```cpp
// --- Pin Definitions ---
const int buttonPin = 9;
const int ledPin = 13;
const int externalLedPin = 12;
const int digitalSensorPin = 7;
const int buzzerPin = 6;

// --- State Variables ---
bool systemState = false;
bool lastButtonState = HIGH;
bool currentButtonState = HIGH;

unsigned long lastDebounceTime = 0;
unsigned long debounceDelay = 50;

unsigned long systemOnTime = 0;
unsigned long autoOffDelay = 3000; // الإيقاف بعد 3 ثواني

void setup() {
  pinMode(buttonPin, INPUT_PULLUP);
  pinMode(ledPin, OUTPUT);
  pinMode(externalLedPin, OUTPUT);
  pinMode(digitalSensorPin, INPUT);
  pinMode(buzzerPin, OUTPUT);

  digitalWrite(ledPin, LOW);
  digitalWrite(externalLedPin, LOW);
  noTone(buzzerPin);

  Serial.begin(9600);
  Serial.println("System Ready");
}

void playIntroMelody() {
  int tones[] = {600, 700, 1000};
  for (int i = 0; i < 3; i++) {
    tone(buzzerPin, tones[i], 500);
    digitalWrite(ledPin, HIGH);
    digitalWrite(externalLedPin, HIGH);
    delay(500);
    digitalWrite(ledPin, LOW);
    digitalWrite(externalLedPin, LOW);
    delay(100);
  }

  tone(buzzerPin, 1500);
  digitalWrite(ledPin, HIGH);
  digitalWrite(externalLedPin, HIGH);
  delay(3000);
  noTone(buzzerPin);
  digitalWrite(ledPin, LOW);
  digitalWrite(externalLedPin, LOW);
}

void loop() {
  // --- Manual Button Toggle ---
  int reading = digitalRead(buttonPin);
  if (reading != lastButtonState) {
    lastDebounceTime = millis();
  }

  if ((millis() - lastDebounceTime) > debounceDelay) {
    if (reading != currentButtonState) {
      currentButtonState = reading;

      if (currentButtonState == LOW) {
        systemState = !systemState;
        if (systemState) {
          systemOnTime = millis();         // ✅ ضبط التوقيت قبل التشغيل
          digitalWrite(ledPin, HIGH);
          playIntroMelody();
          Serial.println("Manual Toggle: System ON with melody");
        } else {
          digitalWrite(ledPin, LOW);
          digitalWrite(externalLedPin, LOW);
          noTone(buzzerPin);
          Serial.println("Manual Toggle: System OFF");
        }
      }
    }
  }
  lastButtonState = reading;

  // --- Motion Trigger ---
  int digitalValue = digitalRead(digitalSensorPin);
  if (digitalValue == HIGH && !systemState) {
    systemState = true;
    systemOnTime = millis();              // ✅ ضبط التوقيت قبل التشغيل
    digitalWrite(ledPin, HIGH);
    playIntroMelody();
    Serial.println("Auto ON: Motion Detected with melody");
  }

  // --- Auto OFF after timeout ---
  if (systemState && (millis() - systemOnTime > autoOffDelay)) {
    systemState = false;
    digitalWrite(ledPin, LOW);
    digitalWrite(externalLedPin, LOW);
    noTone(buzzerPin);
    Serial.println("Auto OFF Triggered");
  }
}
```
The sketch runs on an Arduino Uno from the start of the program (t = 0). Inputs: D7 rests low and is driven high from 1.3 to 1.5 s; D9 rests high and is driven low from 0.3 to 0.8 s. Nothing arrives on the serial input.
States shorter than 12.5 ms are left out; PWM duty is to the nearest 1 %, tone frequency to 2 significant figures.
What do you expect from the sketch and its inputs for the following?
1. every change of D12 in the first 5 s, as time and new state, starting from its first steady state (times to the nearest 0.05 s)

0 s low; 0.35 s high; 0.85 s low; 0.95 s high; 1.45 s low; 1.55 s high; 2.05 s low; 2.15 s high
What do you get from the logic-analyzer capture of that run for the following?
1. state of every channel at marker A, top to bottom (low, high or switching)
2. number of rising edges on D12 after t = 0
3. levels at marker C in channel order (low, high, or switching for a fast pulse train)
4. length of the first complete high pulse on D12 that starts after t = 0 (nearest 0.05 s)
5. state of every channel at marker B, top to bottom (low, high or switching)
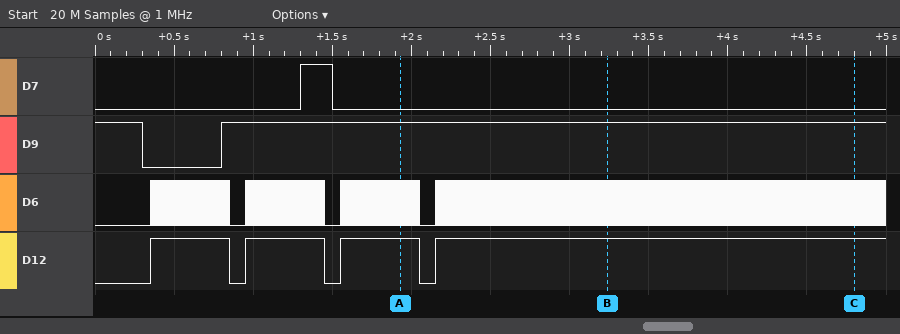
D7 low, D9 high, D6 switching, D12 high
4
D7 low, D9 high, D6 switching, D12 high
0.50 s
D7 low, D9 high, D6 switching, D12 high
